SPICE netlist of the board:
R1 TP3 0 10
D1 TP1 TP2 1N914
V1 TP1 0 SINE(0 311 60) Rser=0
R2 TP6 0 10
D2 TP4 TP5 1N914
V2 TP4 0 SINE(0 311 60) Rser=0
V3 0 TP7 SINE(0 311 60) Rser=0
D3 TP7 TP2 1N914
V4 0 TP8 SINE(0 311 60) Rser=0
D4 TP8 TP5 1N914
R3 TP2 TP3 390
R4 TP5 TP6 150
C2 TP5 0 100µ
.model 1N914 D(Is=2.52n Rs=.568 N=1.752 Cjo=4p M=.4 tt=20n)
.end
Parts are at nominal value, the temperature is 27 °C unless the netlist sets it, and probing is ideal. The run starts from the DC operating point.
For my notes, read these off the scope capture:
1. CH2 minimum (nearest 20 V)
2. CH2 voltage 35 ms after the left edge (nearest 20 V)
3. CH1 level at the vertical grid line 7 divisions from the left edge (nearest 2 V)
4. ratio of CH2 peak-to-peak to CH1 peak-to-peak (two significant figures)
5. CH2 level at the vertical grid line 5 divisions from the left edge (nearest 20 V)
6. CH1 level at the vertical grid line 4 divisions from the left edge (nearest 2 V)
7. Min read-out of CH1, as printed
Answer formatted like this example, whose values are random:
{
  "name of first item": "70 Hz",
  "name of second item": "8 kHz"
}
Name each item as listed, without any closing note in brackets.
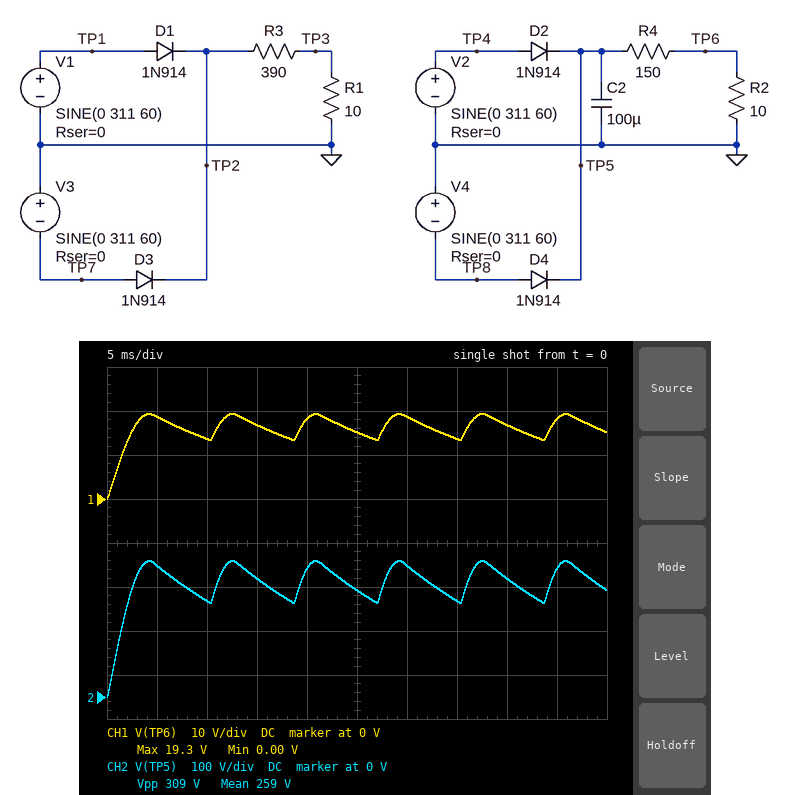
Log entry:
{
  "CH2 minimum": "0 V",
  "CH2 voltage 35 ms after the left edge": "220 V",
  "CH1 level at the vertical grid line 7 divisions from the left edge": "14 V",
  "ratio of CH2 peak-to-peak to CH1 peak-to-peak": "16",
  "CH2 level at the vertical grid line 5 divisions from the left edge": "240 V",
  "CH1 level at the vertical grid line 4 divisions from the left edge": "18 V",
  "Min read-out of CH1, as printed": "0.00 V"
}
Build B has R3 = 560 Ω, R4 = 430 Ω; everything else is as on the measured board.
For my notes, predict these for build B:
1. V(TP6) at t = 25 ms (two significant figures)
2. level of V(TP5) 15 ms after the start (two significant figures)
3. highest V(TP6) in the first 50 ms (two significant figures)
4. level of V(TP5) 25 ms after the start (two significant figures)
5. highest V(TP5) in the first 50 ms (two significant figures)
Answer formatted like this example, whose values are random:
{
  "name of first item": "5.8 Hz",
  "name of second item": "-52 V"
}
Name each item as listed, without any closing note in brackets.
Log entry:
{
  "V(TP6) at t = 25 ms": "6.4 V",
  "level of V(TP5) 15 ms after the start": "290 V",
  "highest V(TP6) in the first 50 ms": "7.0 V",
  "level of V(TP5) 25 ms after the start": "280 V",
  "highest V(TP5) in the first 50 ms": "310 V"
}
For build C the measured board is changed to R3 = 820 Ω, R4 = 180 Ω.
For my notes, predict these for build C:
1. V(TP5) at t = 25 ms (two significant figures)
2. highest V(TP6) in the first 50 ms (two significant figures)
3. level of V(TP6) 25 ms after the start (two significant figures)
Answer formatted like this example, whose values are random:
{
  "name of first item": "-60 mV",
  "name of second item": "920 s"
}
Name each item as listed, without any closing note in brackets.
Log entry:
{
  "V(TP5) at t = 25 ms": "250 V",
  "highest V(TP6) in the first 50 ms": "16 V",
  "level of V(TP6) 25 ms after the start": "13 V"
}
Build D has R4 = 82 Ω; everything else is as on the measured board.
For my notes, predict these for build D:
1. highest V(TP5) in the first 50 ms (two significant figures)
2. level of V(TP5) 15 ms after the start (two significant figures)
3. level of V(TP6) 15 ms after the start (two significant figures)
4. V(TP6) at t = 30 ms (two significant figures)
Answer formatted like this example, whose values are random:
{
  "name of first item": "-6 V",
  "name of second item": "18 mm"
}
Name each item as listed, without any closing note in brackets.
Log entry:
{
  "highest V(TP5) in the first 50 ms": "310 V",
  "level of V(TP5) 15 ms after the start": "250 V",
  "level of V(TP6) 15 ms after the start": "27 V",
  "V(TP6) at t = 30 ms": "32 V"
}
